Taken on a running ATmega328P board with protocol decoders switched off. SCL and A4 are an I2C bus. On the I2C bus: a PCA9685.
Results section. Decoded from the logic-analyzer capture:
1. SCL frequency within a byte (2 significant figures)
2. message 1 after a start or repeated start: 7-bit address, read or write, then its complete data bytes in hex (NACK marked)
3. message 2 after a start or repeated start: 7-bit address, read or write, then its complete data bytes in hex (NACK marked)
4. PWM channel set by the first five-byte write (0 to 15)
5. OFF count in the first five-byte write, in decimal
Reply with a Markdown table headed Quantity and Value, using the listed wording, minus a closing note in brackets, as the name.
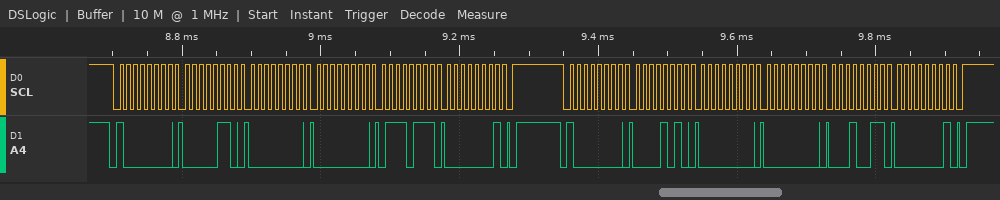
| Quantity | Value |
|---|---|
| SCL frequency within a byte | 100 kHz |
| message 1 after a start or repeated start: 7-bit address, read or write, then its complete data bytes in hex | 0x40 write: 06 00 00 77 01 |
| message 2 after a start or repeated start: 7-bit address, read or write, then its complete data bytes in hex | 0x40 write: 0A 00 00 13 01 |
| PWM channel set by the first five-byte write | 0 |
| OFF count in the first five-byte write, in decimal | 375 |
